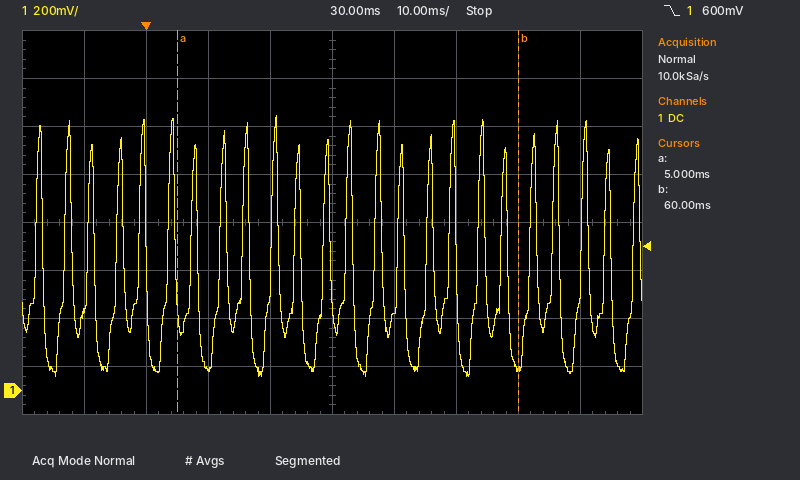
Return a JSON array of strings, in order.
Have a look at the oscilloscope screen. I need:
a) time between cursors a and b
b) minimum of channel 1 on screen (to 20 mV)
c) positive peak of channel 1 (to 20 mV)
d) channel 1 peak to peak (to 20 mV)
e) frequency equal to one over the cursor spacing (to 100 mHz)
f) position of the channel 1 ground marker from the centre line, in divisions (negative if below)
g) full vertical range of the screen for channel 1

["55 ms", "60 mV", "1.14 V", "1.08 V", "18.2 Hz", "-3.5 div", "1.6 V"]
